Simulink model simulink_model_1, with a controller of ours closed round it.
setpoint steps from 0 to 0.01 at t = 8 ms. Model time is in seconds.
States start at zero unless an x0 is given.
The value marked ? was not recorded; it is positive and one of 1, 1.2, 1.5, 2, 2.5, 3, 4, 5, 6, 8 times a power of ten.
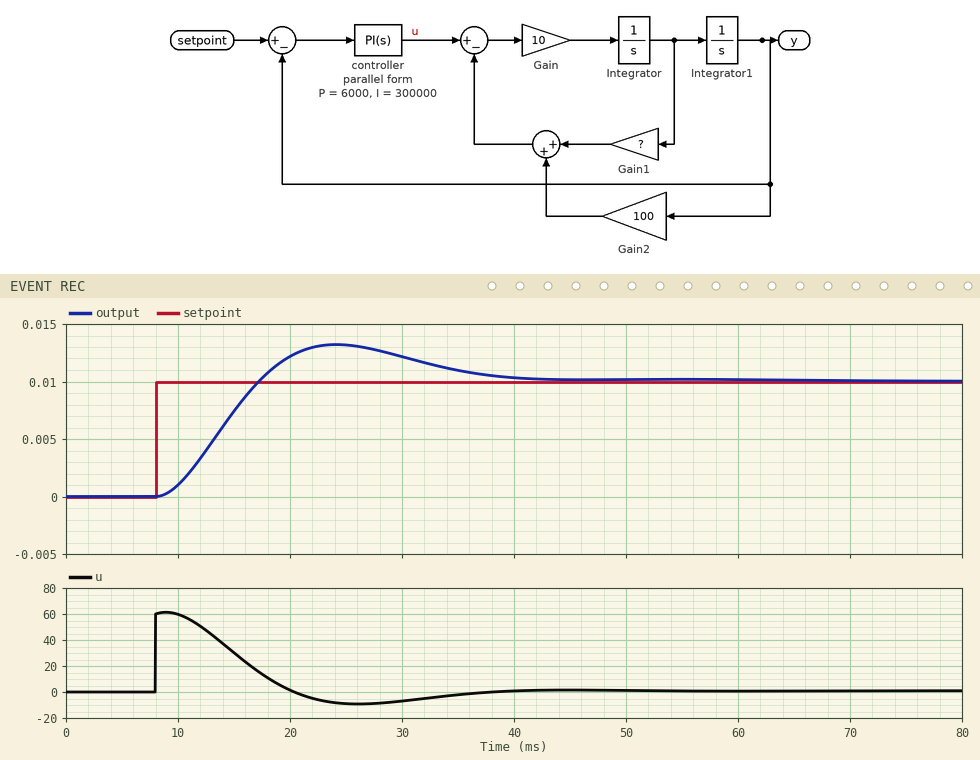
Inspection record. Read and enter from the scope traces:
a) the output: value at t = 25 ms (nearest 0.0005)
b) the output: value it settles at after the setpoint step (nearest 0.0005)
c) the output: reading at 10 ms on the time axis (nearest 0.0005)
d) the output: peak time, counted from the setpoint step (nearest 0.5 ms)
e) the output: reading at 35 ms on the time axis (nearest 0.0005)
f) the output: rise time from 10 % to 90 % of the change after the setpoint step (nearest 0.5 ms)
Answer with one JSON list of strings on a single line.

["0.0130", "0.0100", "0.0010", "16.0 ms", "0.0110", "6.5 ms"]
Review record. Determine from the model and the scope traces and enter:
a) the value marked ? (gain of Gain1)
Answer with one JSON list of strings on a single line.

["30"]
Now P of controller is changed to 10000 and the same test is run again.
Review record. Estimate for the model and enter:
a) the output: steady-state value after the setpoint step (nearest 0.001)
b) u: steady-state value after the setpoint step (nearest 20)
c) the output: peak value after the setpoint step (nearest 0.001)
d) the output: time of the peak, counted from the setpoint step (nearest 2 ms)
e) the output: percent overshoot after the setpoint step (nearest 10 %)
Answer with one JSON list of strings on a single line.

["0.010", "0", "0.013", "12 ms", "30 %"]
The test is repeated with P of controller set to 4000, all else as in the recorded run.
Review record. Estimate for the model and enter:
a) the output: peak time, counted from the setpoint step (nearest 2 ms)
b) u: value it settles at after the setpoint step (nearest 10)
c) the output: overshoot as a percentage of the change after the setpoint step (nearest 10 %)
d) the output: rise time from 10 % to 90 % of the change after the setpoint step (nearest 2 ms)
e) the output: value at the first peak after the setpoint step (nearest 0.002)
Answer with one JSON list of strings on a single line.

["20 ms", "0", "40 %", "8 ms", "0.014"]
